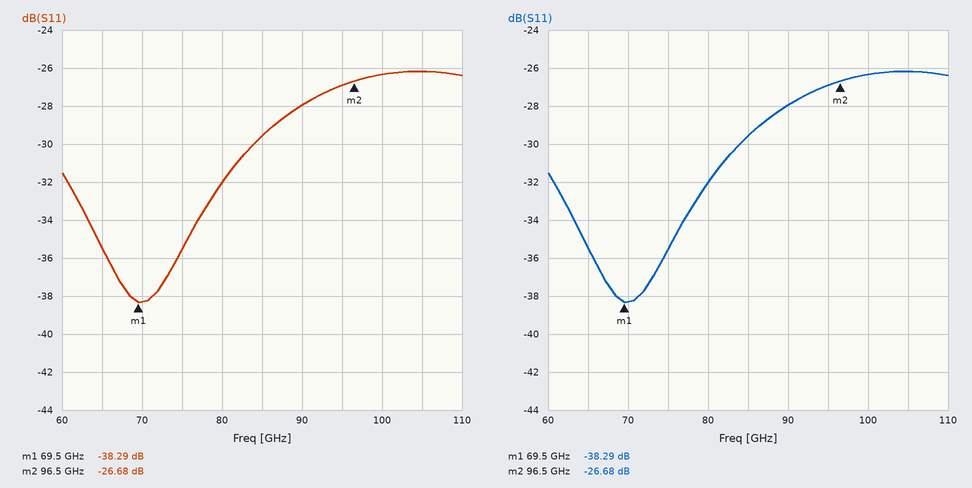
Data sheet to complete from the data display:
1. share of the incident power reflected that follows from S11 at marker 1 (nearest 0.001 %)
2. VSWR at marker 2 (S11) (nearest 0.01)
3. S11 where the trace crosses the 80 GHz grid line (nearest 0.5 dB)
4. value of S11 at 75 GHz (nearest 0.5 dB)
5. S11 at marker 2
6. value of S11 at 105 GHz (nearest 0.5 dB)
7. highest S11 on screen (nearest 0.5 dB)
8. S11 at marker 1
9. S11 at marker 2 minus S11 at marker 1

0.015 %
1.10
-32.0 dB
-35.5 dB
-26.68 dB
-26.0 dB
-26.0 dB
-38.29 dB
11.61 dB
